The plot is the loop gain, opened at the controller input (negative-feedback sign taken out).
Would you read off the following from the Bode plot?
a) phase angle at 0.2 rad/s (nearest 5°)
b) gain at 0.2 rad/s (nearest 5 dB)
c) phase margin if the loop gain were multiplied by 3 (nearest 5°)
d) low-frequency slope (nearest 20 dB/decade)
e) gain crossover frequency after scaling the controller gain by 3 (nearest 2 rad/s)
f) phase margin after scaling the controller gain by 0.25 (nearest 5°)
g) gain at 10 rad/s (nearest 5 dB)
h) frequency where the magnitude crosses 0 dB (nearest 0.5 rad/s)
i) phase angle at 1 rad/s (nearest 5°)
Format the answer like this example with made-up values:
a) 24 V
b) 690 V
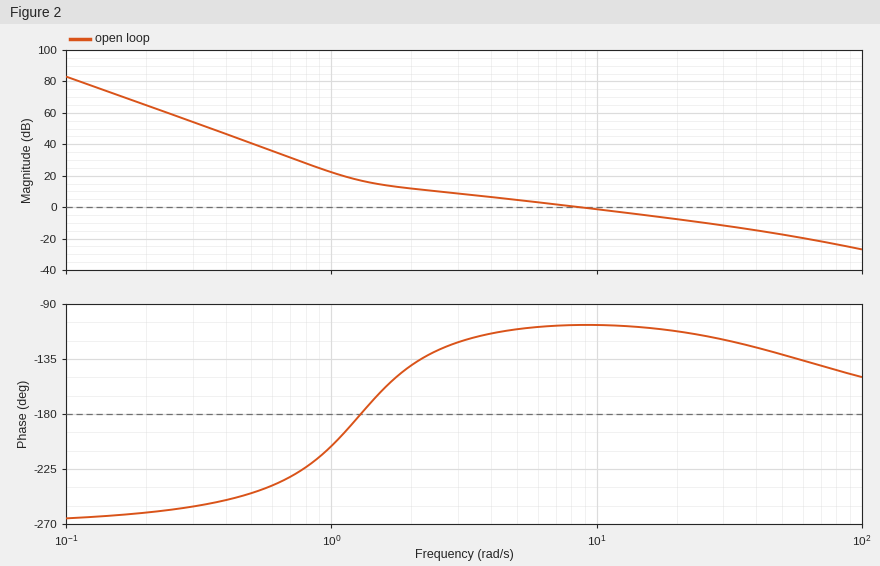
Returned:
a) -260°
b) 65 dB
c) 65°
d) -60 dB/decade
e) 24 rad/s
f) 40°
g) 0 dB
h) 8.5 rad/s
i) -205°
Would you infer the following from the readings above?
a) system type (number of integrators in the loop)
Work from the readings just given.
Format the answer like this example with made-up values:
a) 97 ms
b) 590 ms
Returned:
a) 3
